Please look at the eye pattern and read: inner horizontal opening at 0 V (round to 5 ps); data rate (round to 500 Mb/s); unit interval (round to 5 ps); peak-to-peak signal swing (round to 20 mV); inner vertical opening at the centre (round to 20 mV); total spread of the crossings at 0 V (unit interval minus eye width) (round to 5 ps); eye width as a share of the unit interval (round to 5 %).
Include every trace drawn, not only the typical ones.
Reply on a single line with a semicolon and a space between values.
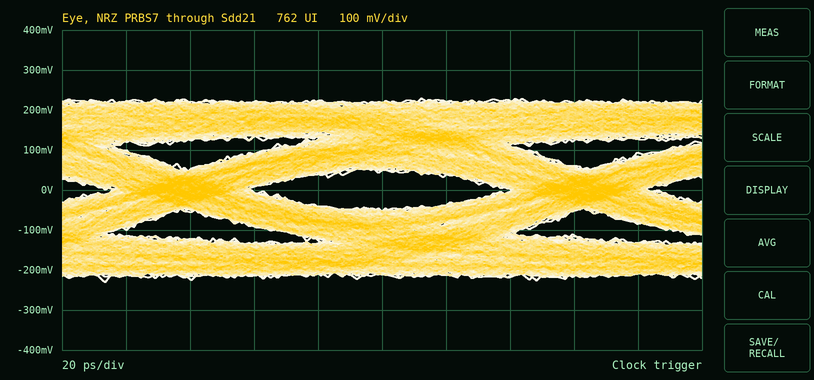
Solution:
80 ps; 8.0 Gb/s; 125 ps; 460 mV; 100 mV; 45 ps; 65 %
